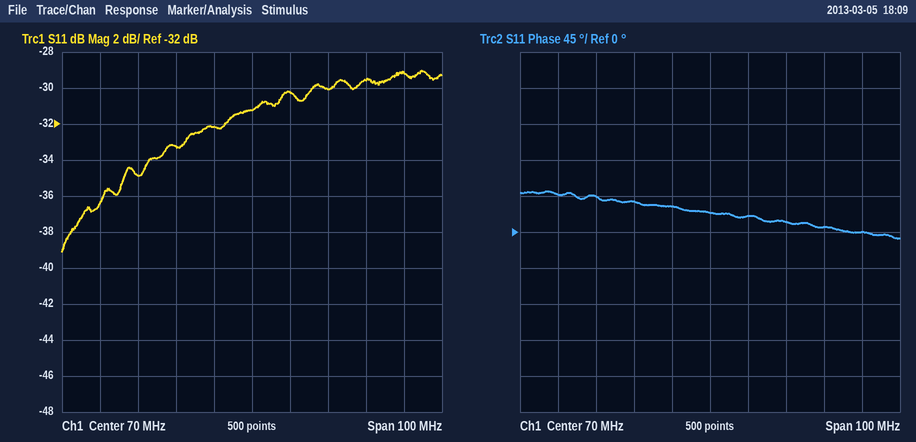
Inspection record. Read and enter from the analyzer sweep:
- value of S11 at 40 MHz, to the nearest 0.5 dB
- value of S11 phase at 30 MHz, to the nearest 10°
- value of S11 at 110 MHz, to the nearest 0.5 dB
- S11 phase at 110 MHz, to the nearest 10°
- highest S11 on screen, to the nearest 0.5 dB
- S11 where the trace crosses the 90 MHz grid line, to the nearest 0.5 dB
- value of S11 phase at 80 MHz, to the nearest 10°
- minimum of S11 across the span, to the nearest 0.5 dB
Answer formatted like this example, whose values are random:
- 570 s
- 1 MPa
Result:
- -35.0 dB
- 50°
- -29.0 dB
- 0°
- -29.0 dB
- -30.0 dB
- 20°
- -39.0 dB
